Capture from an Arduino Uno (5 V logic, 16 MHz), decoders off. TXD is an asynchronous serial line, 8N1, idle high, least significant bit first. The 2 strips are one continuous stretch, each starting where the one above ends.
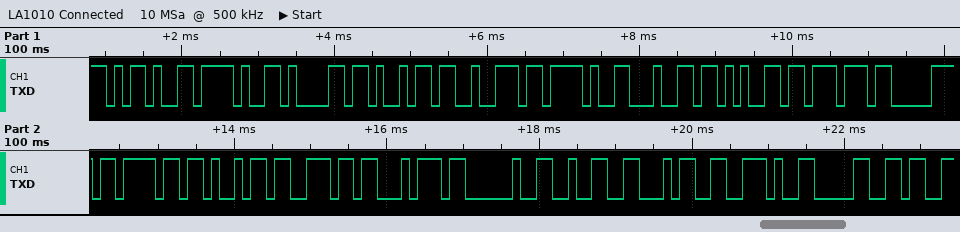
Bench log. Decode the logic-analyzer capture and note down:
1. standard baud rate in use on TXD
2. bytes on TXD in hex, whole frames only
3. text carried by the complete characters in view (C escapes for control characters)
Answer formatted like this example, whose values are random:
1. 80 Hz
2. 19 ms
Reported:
1. 9600 baud
2. 2D 2F 61 69 72 2F 64 65 77 70 6F 69 6E 74 20 32 34 2E 30
3. "-/air/dewpoint 24.0"
